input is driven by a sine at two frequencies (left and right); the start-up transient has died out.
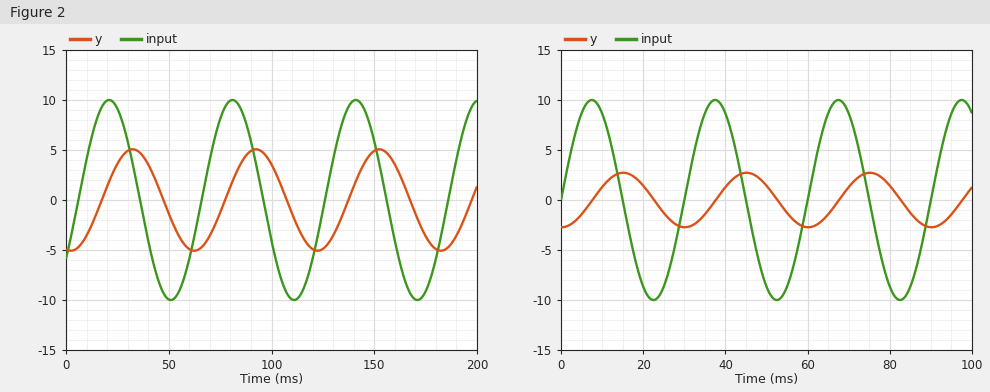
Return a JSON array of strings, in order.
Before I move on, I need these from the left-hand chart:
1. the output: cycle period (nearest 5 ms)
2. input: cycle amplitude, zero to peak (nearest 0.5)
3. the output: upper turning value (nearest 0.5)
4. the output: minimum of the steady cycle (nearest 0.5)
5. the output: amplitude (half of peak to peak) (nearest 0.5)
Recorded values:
["60 ms", "10.0", "5.0", "-5.0", "5.0"]
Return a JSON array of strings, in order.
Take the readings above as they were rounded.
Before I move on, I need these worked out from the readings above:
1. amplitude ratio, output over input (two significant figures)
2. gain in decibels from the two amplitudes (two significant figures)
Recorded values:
["0.50", "-6.0 dB"]
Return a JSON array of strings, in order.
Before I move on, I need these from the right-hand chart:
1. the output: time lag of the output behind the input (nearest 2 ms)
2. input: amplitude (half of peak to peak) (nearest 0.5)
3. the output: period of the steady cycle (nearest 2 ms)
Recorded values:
["8 ms", "10.0", "30 ms"]
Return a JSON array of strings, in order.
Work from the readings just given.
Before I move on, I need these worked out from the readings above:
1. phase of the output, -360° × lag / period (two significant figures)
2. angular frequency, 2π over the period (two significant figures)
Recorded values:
["-96°", "0.21 rad/ms"]
